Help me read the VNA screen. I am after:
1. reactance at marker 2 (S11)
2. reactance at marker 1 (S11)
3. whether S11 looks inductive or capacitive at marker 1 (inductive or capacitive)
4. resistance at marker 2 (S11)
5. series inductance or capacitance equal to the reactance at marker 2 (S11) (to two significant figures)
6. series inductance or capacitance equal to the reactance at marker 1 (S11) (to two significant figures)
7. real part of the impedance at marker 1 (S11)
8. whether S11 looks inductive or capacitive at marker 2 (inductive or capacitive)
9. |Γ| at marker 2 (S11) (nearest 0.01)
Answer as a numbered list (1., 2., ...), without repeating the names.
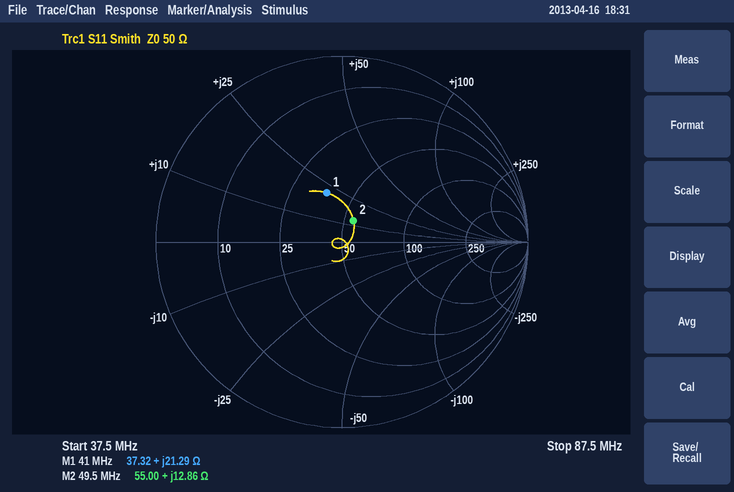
1. +12.86 Ω
2. +21.29 Ω
3. inductive
4. 55.00 Ω
5. 41 nH
6. 83 nH
7. 37.32 Ω
8. inductive
9. 0.13
